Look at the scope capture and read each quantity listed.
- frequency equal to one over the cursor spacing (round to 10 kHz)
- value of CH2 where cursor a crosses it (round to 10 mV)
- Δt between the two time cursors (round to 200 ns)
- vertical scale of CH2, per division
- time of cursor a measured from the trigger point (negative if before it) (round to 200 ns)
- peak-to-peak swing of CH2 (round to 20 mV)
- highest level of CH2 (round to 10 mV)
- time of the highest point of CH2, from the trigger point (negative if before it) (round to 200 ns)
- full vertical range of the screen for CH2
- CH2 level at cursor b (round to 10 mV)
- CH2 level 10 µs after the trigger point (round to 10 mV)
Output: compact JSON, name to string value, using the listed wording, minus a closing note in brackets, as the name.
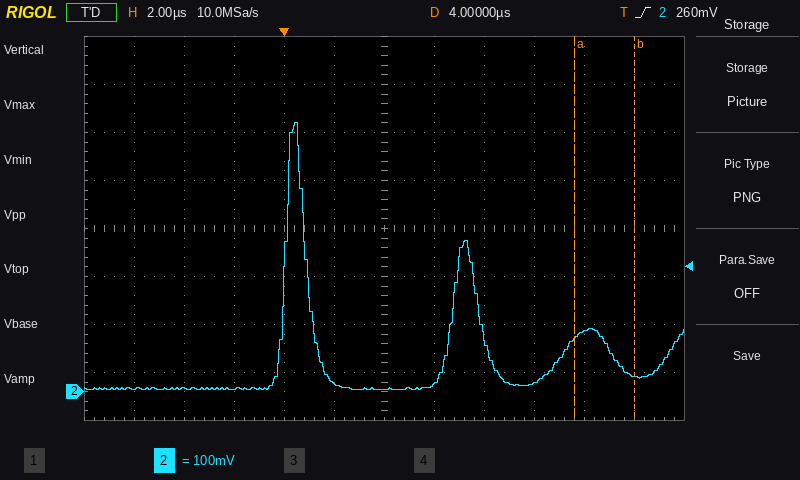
{"frequency equal to one over the cursor spacing": "420 kHz", "value of CH2 where cursor a crosses it": "110 mV", "Δt between the two time cursors": "2.4 µs", "vertical scale of CH2, per division": "100 mV", "time of cursor a measured from the trigger point (negative if before it)": "+11.6 µs", "peak-to-peak swing of CH2": "560 mV", "highest level of CH2": "560 mV", "time of the highest point of CH2, from the trigger point (negative if before it)": "+400 ns", "full vertical range of the screen for CH2": "800 mV", "CH2 level at cursor b": "30 mV", "CH2 level 10 µs after the trigger point": "20 mV"}
